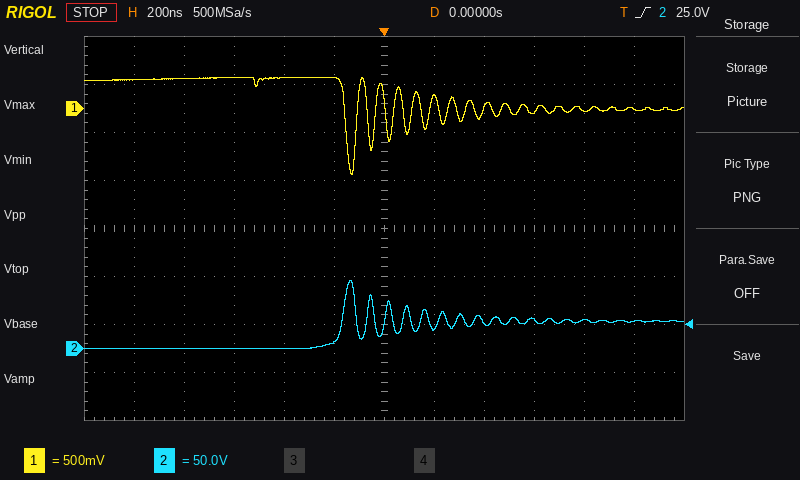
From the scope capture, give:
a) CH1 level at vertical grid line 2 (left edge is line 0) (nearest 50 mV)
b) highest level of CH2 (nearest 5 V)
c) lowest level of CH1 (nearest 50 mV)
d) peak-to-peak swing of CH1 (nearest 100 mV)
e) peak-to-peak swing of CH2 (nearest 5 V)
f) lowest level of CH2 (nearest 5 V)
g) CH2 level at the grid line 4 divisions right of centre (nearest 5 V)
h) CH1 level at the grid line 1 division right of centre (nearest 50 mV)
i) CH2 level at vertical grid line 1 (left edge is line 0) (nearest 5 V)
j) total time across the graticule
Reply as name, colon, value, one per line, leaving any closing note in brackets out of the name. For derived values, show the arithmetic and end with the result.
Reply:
CH1 level at vertical grid line 2 (left edge is line 0): 300 mV
highest level of CH2: 70 V
lowest level of CH1: -700 mV
peak-to-peak swing of CH1: 1.00 V
peak-to-peak swing of CH2: 70 V − (0 V) = 70 V
lowest level of CH2: 0 V
CH2 level at the grid line 4 divisions right of centre: 30 V
CH1 level at the grid line 1 division right of centre: 100 mV
CH2 level at vertical grid line 1 (left edge is line 0): 0 V
total time across the graticule: 2.4 µs
